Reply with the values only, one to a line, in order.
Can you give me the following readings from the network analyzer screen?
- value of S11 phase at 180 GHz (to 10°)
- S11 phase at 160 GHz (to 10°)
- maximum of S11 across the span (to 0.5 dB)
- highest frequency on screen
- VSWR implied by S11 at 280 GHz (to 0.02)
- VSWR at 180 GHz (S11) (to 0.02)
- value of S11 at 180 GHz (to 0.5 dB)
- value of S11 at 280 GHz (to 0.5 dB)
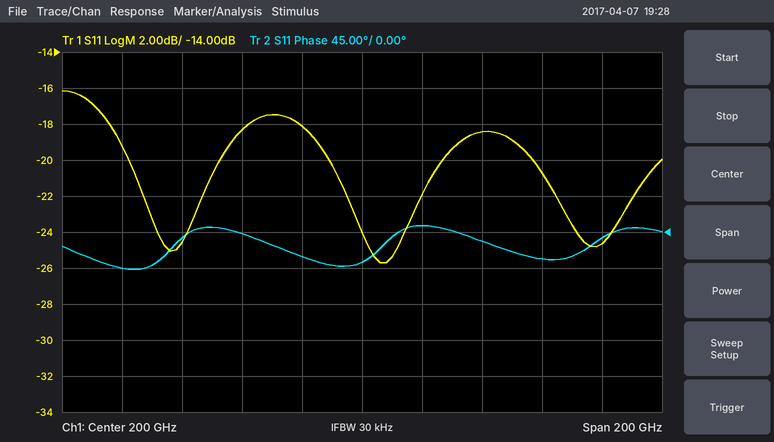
-30°
0°
-16.0 dB
300 GHz
1.12
1.28
-18.0 dB
-24.5 dB
